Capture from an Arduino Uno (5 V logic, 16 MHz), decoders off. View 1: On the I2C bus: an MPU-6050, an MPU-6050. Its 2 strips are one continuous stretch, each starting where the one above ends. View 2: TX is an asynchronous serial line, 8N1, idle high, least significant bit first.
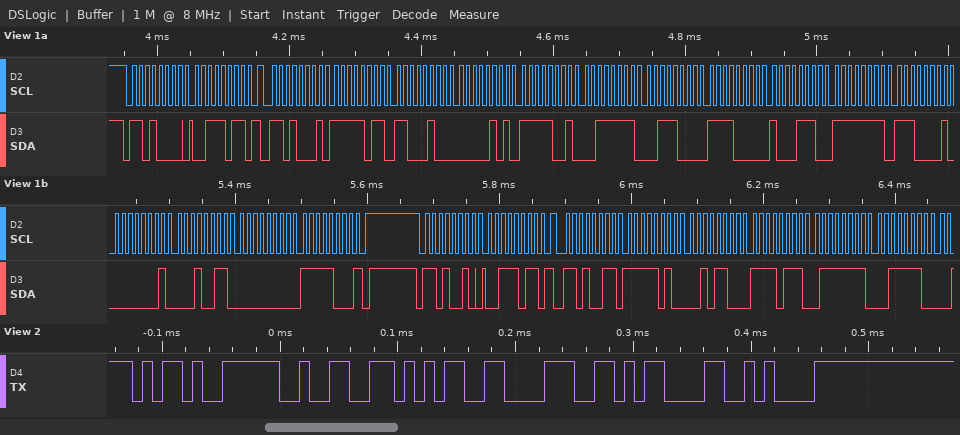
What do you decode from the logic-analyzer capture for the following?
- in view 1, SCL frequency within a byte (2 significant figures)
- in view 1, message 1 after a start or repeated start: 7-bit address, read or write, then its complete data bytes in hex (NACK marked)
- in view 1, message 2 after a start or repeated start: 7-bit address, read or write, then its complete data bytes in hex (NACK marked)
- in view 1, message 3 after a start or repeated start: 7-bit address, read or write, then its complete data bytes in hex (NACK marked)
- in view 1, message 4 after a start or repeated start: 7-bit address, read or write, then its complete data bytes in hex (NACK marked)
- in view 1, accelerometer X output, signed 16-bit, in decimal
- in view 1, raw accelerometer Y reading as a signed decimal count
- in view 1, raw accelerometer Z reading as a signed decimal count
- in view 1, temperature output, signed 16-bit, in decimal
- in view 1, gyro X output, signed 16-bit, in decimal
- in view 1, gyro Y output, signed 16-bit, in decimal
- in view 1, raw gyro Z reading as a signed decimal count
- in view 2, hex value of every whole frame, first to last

100 kHz
0x68 write: 3B
0x68 read: FB C4 05 F9 3F 38 F0 8E FF E1 01 13 00 F8 NACK
0x69 write: 3B
0x69 read: FA 2C F7 7F 3E
-1084
1529
16184
-3954
-31
275
248
2D 32 35 38 0D 0A
